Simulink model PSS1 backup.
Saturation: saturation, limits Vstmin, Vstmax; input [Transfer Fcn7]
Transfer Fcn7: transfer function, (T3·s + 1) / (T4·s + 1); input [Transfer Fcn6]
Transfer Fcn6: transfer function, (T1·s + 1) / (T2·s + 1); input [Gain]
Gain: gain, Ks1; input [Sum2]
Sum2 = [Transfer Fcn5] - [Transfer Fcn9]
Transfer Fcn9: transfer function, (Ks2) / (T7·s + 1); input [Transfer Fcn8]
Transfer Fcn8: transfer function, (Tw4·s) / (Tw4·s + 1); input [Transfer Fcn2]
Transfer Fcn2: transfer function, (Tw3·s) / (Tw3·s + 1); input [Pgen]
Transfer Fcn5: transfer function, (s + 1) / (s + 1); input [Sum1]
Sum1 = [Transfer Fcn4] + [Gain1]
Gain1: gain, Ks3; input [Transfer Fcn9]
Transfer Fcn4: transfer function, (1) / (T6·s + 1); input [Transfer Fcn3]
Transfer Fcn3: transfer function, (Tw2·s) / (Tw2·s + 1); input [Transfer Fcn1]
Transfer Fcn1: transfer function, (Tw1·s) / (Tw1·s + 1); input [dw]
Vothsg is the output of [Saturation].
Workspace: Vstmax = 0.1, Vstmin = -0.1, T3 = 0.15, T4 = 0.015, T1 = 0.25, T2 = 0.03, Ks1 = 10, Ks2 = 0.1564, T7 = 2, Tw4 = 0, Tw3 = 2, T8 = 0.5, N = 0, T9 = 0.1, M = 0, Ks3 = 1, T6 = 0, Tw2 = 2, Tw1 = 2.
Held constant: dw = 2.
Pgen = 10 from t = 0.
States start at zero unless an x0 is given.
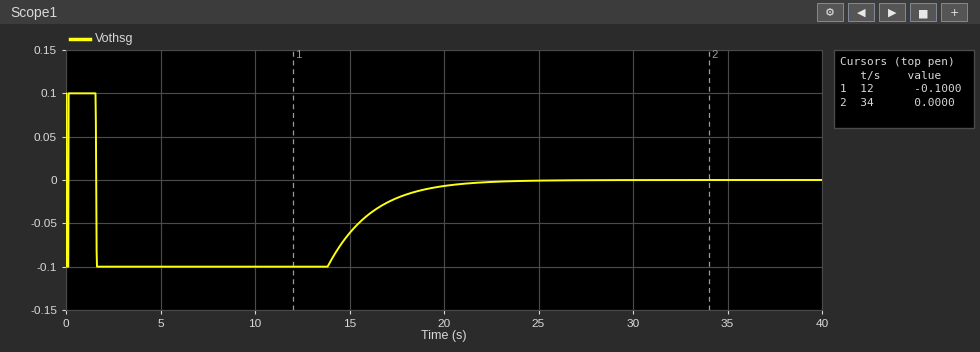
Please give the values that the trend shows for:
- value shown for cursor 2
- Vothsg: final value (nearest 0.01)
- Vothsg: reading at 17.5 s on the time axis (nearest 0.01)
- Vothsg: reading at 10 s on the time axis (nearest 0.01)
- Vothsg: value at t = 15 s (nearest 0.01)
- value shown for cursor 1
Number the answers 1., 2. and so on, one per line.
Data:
1. 0.0000
2. 0.00
3. -0.02
4. -0.10
5. -0.06
6. -0.1000
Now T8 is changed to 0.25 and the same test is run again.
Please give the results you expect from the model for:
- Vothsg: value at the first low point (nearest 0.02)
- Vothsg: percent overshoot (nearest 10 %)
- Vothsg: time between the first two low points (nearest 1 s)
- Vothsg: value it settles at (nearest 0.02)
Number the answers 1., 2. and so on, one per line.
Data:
1. -0.10
2. 100 %
3. 8 s
4. 0.00
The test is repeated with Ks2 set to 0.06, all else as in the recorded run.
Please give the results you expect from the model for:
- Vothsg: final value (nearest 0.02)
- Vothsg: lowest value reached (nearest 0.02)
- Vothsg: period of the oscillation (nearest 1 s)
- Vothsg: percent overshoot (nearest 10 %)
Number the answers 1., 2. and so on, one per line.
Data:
1. 0.00
2. -0.10
3. 8 s
4. 100 %
